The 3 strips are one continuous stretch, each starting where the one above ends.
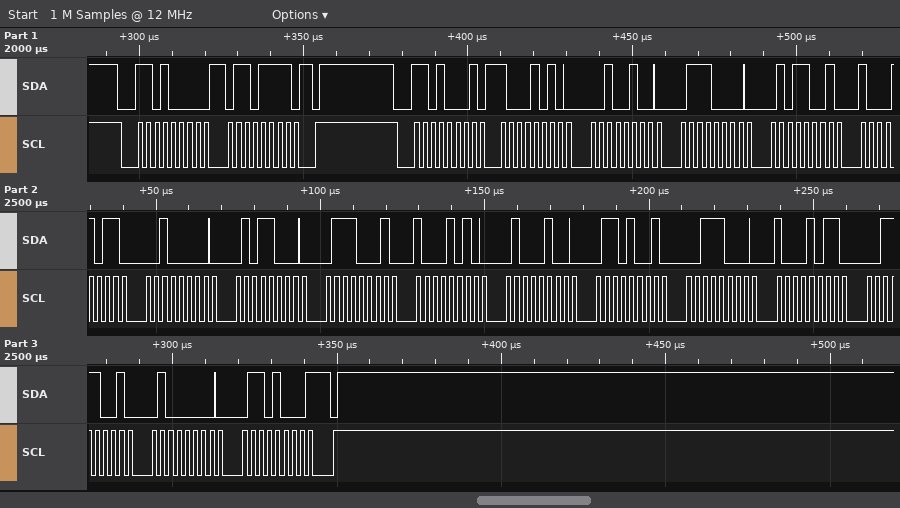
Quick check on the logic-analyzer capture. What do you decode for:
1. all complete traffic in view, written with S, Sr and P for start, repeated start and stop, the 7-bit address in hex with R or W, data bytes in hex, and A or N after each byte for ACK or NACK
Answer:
S 68W A 6F A P S 68R A 8A A 24 A 70 A 59 A 8B A 20 A 58 A 71 A 8A A 44 A 69 A 38 A 8B A 39 A 40 A 68 N P
